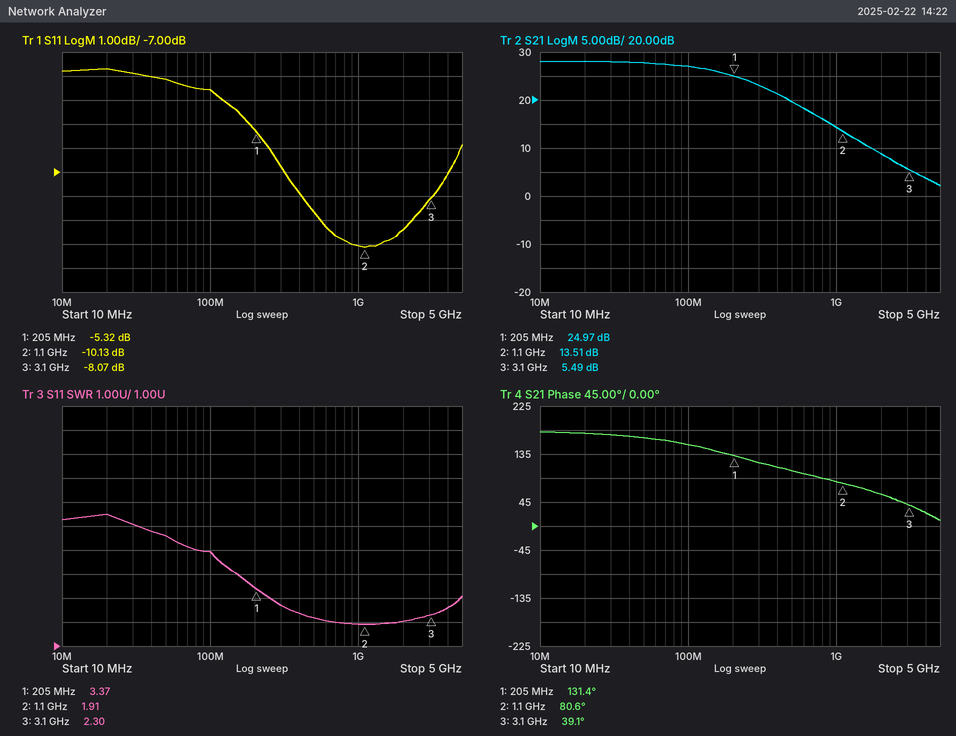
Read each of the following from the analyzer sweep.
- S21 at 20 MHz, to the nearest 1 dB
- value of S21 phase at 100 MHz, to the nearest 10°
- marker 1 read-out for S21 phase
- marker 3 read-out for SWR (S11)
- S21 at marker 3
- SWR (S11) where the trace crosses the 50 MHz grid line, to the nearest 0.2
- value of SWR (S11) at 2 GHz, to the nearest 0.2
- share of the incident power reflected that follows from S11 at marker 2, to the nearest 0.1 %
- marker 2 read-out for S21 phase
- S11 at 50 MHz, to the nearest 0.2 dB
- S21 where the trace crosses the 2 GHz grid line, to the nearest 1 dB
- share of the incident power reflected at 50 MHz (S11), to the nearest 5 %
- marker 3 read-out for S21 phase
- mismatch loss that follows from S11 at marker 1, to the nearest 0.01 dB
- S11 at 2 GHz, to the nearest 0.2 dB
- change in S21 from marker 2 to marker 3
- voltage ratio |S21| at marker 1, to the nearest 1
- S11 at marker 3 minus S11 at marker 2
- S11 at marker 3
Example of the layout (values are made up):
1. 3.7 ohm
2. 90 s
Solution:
1. 28 dB
2. 150°
3. 131.4°
4. 2.30
5. 5.49 dB
6. 5.6
7. 2.0
8. 9.7 %
9. 80.6°
10. -3.2 dB
11. 9 dB
12. 50 %
13. 39.1°
14. 1.51 dB
15. -9.4 dB
16. -8.02 dB
17. 18
18. 2.06 dB
19. -8.07 dB
